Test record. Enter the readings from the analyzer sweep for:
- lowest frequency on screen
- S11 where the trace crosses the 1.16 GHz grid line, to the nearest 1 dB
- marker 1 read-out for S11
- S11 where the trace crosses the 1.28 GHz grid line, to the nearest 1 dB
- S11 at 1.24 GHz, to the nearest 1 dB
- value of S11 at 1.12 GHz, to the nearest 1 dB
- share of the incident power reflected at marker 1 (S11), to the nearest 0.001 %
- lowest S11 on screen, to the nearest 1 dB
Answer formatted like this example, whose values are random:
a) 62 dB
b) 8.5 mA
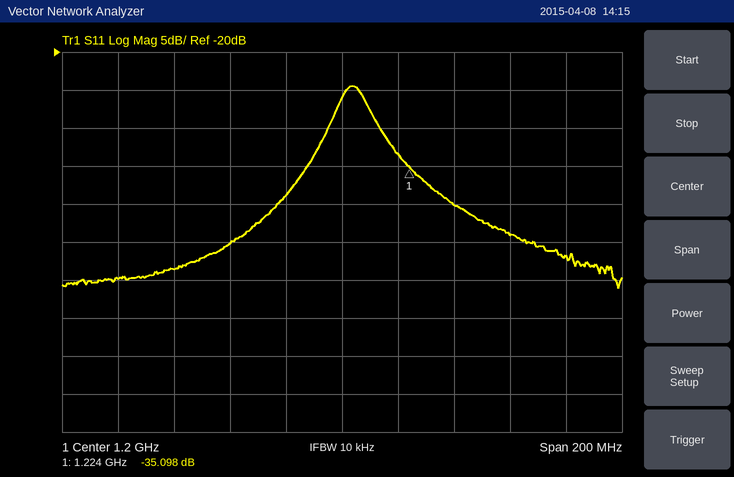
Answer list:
a) 1.1 GHz
b) -45 dB
c) -35.098 dB
d) -47 dB
e) -40 dB
f) -50 dB
g) 0.031 %
h) -51 dB
